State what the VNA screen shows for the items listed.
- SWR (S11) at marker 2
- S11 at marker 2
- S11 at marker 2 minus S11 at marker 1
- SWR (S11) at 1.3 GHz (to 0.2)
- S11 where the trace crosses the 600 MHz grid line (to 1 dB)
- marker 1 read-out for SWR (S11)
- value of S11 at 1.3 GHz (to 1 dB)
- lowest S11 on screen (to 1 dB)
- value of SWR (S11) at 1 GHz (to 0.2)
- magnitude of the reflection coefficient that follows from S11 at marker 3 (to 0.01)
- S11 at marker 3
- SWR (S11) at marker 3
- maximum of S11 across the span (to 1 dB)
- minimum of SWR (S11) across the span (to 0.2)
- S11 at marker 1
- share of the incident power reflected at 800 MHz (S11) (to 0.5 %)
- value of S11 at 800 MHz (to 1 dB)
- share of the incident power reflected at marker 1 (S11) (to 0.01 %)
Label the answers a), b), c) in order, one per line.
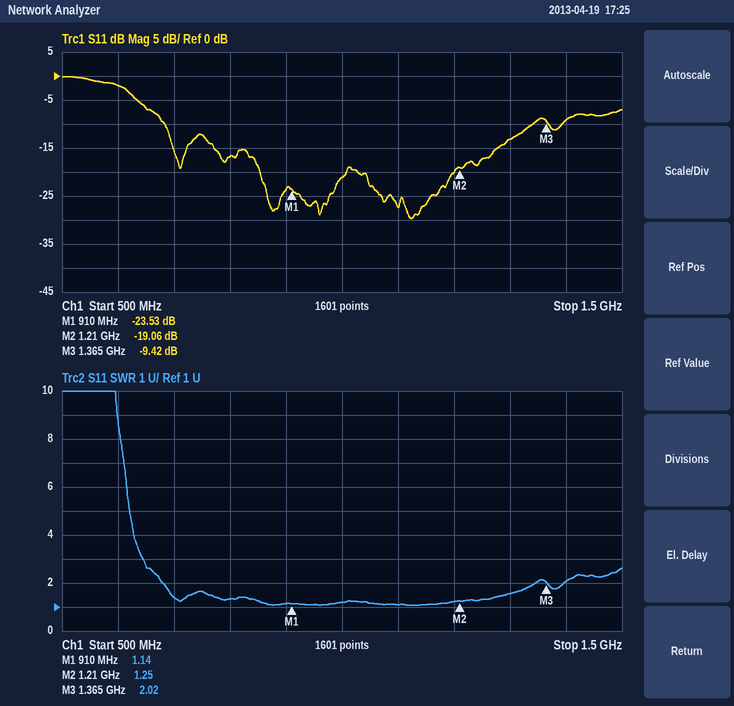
a) 1.25
b) -19.06 dB
c) 4.47 dB
d) 1.6
e) -2 dB
f) 1.14
g) -13 dB
h) -30 dB
i) 1.2
j) 0.34
k) -9.42 dB
l) 2.02
m) 0 dB
n) 1.0
o) -23.53 dB
p) 2.0 %
q) -17 dB
r) 0.44 %
